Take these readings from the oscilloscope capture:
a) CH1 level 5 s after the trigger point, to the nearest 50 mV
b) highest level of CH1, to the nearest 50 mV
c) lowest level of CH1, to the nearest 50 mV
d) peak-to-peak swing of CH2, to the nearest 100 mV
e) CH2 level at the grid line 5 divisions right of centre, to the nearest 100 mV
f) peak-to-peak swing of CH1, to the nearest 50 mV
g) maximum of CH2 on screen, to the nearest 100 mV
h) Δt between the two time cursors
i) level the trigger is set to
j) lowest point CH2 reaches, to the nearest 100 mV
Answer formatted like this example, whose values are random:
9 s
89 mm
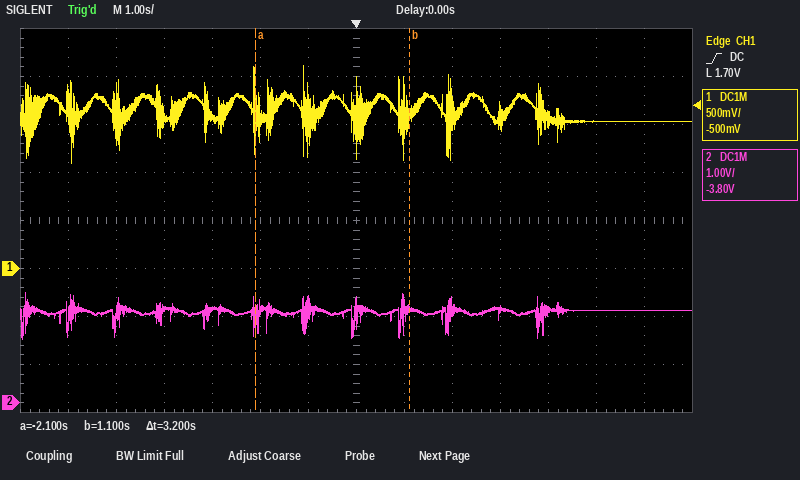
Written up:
1.55 V
2.10 V
1.10 V
1.0 V
1.9 V
1.00 V
2.3 V
3.2 s
1.70 V
1.3 V
